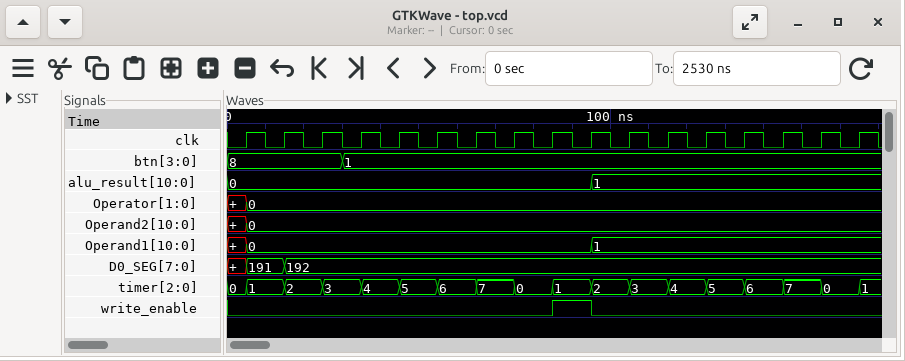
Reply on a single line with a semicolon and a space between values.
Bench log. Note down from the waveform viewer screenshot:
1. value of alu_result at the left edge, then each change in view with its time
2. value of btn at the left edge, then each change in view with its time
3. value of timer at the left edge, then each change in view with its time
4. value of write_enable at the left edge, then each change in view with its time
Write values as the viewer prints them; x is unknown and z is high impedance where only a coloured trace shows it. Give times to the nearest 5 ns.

0, 1 at 95 ns; 8, 1 at 30 ns; 0, 1 at 5 ns, 2 at 15 ns, 3 at 25 ns, 4 at 35 ns, 5 at 45 ns, 6 at 55 ns, 7 at 65 ns, 0 at 75 ns, 1 at 85 ns, 2 at 95 ns, 3 at 105 ns, 4 at 115 ns, 5 at 125 ns, 6 at 135 ns, 7 at 145 ns, 0 at 155 ns, 1 at 165 ns; 0, 1 at 85 ns, 0 at 95 ns
